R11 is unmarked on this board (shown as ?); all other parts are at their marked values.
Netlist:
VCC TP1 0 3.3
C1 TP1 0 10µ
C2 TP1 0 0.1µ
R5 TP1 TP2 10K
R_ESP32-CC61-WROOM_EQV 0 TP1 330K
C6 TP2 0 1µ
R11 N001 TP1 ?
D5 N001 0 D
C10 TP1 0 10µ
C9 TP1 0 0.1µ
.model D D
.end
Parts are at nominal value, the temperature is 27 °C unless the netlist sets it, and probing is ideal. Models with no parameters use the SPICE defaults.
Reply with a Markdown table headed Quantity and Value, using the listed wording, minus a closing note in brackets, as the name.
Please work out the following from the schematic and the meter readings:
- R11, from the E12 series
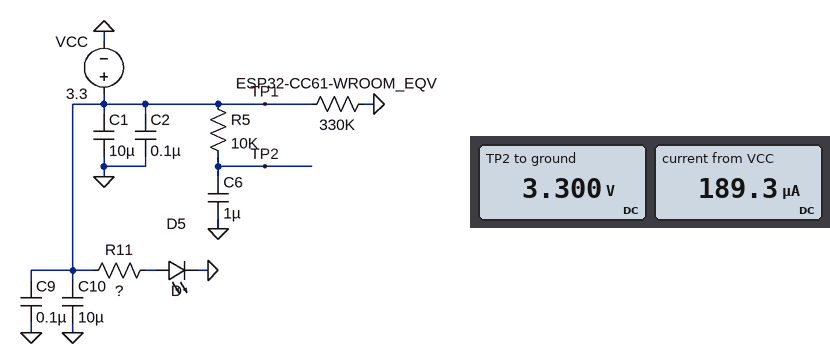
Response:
| Quantity | Value |
|---|---|
| R11, from the E12 series | 15 kΩ |
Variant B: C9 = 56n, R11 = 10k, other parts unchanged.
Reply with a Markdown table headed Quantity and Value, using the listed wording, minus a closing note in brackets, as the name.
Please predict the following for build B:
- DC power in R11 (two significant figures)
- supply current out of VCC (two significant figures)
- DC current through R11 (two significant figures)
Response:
| Quantity | Value |
|---|---|
| DC power in R11 | 720 µW |
| supply current out of VCC | 280 µA |
| DC current through R11 | 270 µA |
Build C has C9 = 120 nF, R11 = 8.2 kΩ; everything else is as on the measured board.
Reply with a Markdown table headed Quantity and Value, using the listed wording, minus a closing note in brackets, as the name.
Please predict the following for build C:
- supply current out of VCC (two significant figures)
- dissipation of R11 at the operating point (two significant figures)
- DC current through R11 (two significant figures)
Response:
| Quantity | Value |
|---|---|
| supply current out of VCC | 340 µA |
| dissipation of R11 at the operating point | 870 µW |
| DC current through R11 | 330 µA |
